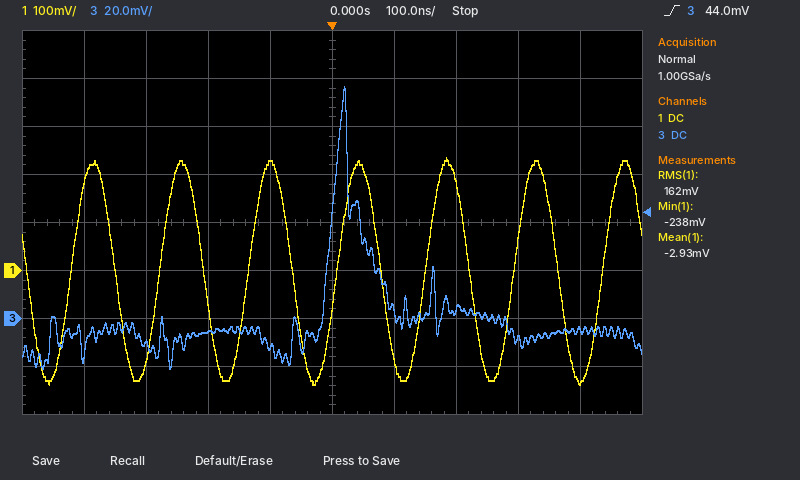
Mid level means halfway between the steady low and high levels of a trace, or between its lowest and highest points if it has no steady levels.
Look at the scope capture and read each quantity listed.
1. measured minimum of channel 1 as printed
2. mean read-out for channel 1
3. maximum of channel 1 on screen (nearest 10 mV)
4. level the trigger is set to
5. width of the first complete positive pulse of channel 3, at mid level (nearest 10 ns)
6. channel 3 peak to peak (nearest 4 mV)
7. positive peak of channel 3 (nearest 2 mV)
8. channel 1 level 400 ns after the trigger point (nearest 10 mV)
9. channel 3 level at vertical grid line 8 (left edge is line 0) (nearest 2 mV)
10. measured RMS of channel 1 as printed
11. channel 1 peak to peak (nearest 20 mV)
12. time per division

-238 mV
-2.93 mV
240 mV
44.0 mV
50 ns
116 mV
96 mV
-230 mV
-10 mV
162 mV
480 mV
100 ns
